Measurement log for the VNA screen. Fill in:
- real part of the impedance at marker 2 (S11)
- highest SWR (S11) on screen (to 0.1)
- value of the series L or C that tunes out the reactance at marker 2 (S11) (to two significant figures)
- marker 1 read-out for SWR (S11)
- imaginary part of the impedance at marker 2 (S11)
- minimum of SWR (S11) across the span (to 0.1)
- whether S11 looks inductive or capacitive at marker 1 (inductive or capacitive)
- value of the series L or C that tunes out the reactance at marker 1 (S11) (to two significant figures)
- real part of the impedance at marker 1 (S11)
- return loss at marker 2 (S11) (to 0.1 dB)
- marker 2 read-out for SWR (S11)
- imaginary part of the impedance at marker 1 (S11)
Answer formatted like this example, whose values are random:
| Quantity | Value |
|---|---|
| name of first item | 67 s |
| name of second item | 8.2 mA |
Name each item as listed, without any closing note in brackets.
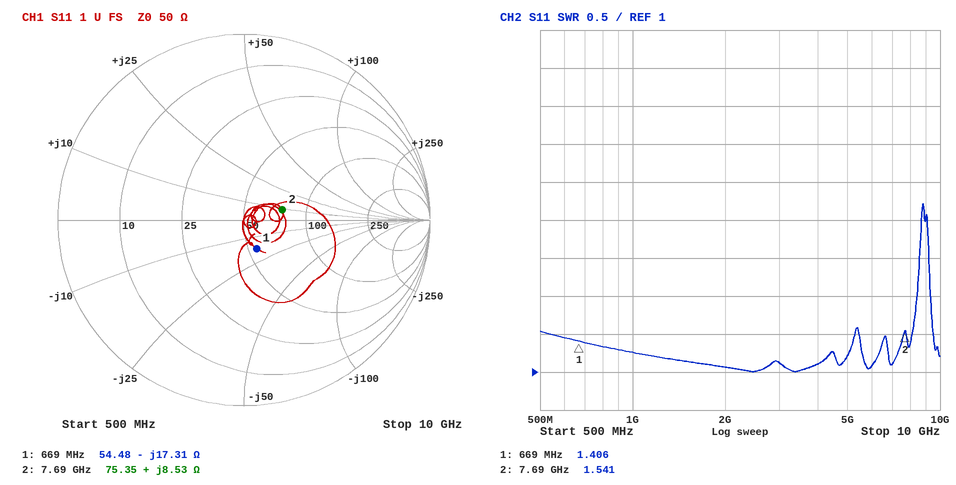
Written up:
| Quantity | Value |
|---|---|
| real part of the impedance at marker 2 | 75.35 Ω |
| highest SWR (S11) on screen | 3.2 |
| value of the series L or C that tunes out the reactance at marker 2 (S11) | 2.4 pF |
| marker 1 read-out for SWR | 1.406 |
| imaginary part of the impedance at marker 2 | +8.53 Ω |
| minimum of SWR (S11) across the span | 1.0 |
| whether S11 looks inductive or capacitive at marker 1 | capacitive |
| value of the series L or C that tunes out the reactance at marker 1 (S11) | 4.1 nH |
| real part of the impedance at marker 1 | 54.48 Ω |
| return loss at marker 2 (S11) | 13.4 dB |
| marker 2 read-out for SWR | 1.541 |
| imaginary part of the impedance at marker 1 | -17.31 Ω |
